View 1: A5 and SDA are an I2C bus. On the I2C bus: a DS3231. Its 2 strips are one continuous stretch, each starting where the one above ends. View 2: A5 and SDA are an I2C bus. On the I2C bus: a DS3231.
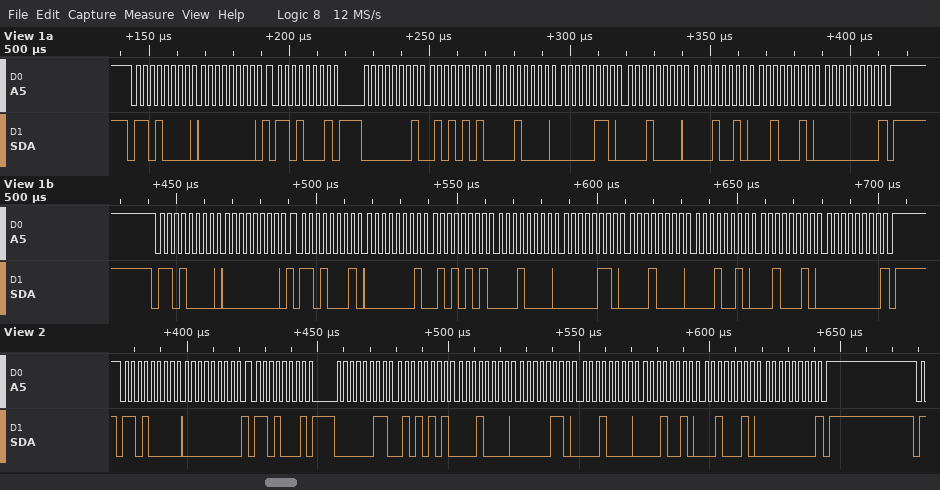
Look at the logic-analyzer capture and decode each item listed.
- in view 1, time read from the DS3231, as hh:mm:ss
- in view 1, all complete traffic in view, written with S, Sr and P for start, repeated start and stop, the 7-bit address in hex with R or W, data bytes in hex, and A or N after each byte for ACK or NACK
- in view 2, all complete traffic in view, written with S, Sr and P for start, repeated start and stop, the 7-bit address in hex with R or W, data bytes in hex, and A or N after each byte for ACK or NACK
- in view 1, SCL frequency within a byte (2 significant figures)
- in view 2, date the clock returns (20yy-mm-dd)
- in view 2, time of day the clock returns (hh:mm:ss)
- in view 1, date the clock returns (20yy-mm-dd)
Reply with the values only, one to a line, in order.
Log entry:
10:55:01
S 68W A 00 A Sr 68R A 01 A 55 A 10 A 06 A 10 A 12 A 22 A 00 N P S 68W A 00 A Sr 68R A 01 A 55 A 10 A 06 A 10 A 12 A 22 A 00 N P
S 68W A 00 A Sr 68R A 03 A 55 A 10 A 06 A 10 A 12 A 22 A 00 N P
400 kHz
2022-12-10
10:55:03
2022-12-10
